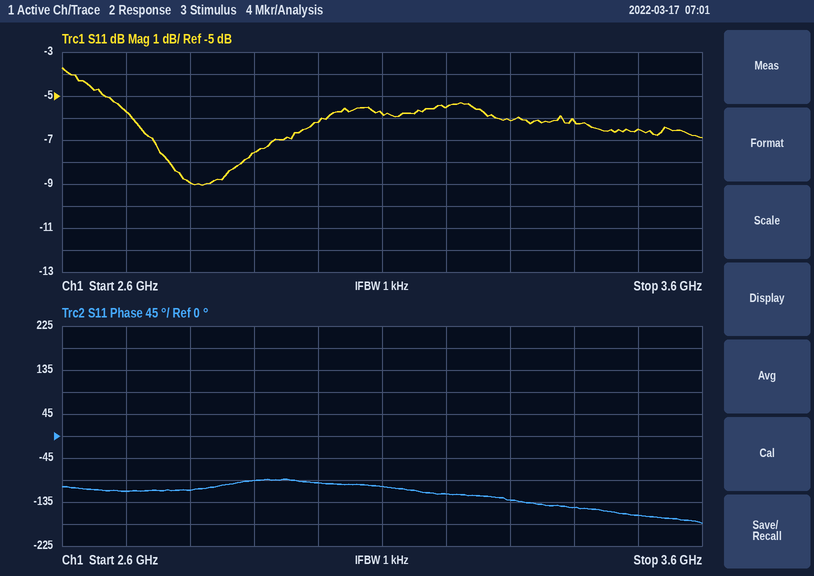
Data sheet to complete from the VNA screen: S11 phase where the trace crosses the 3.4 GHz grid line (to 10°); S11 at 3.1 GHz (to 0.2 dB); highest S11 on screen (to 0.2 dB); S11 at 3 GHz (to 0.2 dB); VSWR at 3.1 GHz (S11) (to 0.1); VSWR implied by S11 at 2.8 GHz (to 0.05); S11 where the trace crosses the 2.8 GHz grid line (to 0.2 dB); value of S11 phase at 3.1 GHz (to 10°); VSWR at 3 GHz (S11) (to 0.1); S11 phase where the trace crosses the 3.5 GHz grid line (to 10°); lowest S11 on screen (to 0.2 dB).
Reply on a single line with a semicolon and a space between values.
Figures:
-150°; -5.8 dB; -3.8 dB; -6.2 dB; 3.1; 2.10; -9.0 dB; -100°; 2.9; -160°; -9.0 dB
